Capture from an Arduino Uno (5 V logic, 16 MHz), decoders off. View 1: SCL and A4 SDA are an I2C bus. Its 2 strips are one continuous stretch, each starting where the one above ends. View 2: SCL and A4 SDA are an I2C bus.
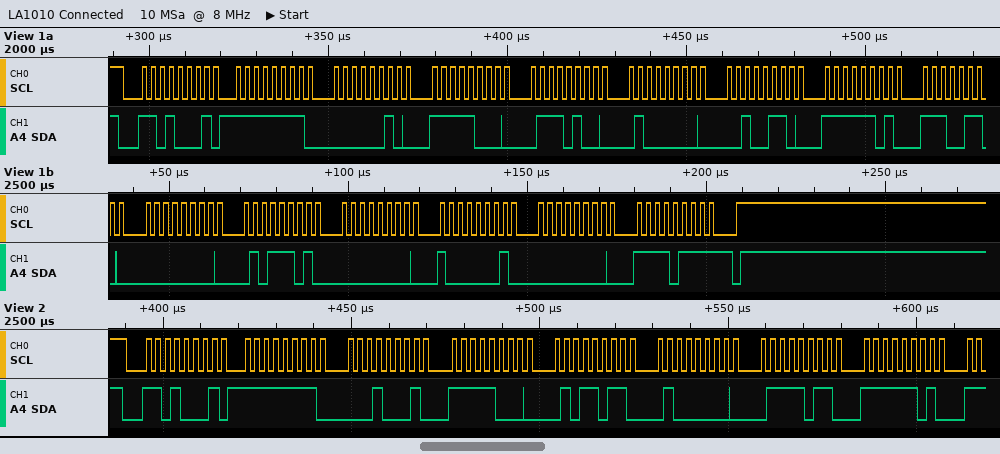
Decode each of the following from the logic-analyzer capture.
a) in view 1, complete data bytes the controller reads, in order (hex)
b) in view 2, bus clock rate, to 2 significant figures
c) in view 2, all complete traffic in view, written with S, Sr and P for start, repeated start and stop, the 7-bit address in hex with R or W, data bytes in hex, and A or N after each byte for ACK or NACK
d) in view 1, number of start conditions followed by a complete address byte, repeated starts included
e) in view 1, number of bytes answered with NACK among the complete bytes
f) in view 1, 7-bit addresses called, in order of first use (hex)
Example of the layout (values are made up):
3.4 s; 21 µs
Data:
FF 02 F8 74 40 26 FD E6 00 5D 00 81 00 F7; 400 kHz; S 68R A FF A 11 A F8 A 5B A 40 A 7B A FD A; 1; 1; 0x68
